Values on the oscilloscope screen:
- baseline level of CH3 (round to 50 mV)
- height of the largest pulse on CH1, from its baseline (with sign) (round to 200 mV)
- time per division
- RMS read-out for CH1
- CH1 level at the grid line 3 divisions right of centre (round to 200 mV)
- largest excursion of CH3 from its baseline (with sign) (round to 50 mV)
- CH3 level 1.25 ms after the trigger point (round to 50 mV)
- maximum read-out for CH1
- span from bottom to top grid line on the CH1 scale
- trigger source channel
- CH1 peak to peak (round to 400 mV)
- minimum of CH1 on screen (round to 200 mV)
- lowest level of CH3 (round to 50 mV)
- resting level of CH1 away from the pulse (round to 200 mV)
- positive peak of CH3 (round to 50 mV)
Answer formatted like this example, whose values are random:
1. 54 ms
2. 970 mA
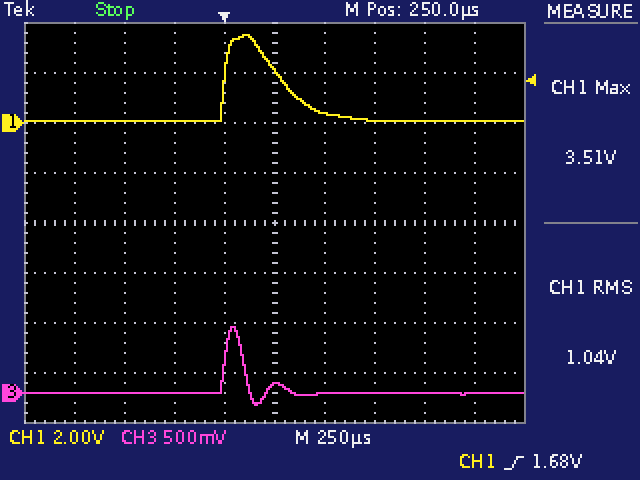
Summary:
1. 0 mV
2. +3.4 V
3. 250 µs
4. 1.04 V
5. 0.0 V
6. +650 mV
7. 0 mV
8. 3.51 V
9. 16 V
10. CH1
11. 3.6 V
12. 0.0 V
13. -100 mV
14. 0.0 V
15. 650 mV
